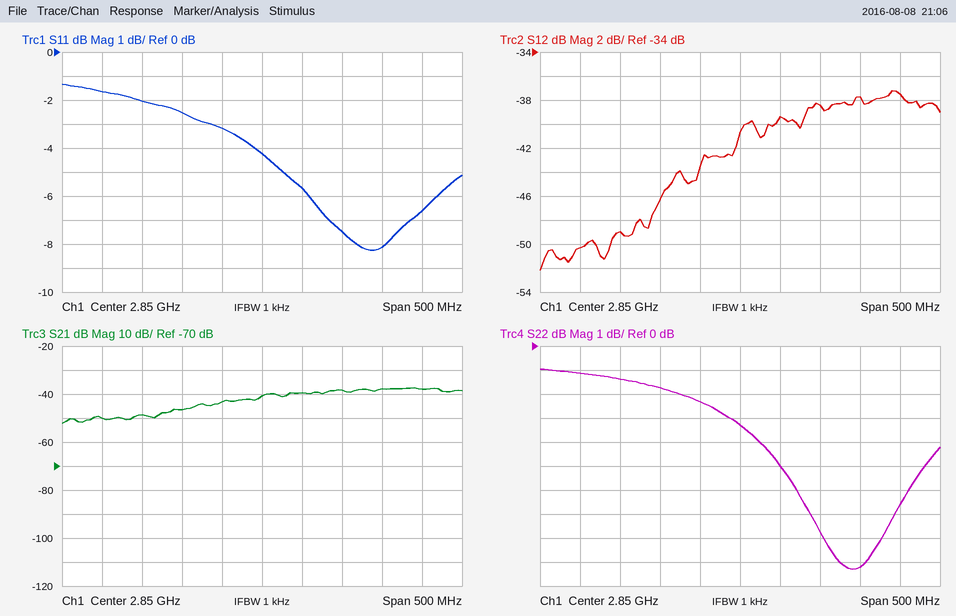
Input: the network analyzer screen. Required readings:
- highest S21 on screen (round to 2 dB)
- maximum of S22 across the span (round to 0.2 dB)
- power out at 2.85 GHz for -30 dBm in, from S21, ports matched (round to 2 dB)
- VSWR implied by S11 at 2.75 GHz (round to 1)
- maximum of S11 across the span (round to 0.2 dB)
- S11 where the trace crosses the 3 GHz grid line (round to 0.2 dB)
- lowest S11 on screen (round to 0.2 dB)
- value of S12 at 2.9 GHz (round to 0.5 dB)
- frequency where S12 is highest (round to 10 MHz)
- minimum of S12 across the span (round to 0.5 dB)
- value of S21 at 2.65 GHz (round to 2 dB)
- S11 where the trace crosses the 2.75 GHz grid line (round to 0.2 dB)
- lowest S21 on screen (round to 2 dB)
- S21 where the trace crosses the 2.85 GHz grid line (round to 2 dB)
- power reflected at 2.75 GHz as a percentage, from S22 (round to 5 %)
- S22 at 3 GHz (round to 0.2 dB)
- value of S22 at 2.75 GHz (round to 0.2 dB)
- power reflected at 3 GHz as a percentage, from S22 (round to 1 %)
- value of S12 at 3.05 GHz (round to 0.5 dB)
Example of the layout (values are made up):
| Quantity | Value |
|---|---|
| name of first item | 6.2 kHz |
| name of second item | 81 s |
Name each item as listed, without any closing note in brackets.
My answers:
| Quantity | Value |
|---|---|
| highest S21 on screen | -38 dB |
| maximum of S22 across the span | -1.0 dB |
| power out at 2.85 GHz for -30 dBm in, from S21, ports matched | -70 dBm |
| VSWR implied by S11 at 2.75 GHz | 7 |
| maximum of S11 across the span | -1.4 dB |
| S11 where the trace crosses the 3 GHz grid line | -8.2 dB |
| lowest S11 on screen | -8.2 dB |
| value of S12 at 2.9 GHz | -39.5 dB |
| frequency where S12 is highest | 3.04 GHz |
| minimum of S12 across the span | -52.0 dB |
| value of S21 at 2.65 GHz | -50 dB |
| S11 where the trace crosses the 2.75 GHz grid line | -2.6 dB |
| lowest S21 on screen | -52 dB |
| S21 where the trace crosses the 2.85 GHz grid line | -40 dB |
| power reflected at 2.75 GHz as a percentage, from S22 | 65 % |
| S22 at 3 GHz | -9.2 dB |
| value of S22 at 2.75 GHz | -1.8 dB |
| power reflected at 3 GHz as a percentage, from S22 | 12 % |
| value of S12 at 3.05 GHz | -37.5 dB |
